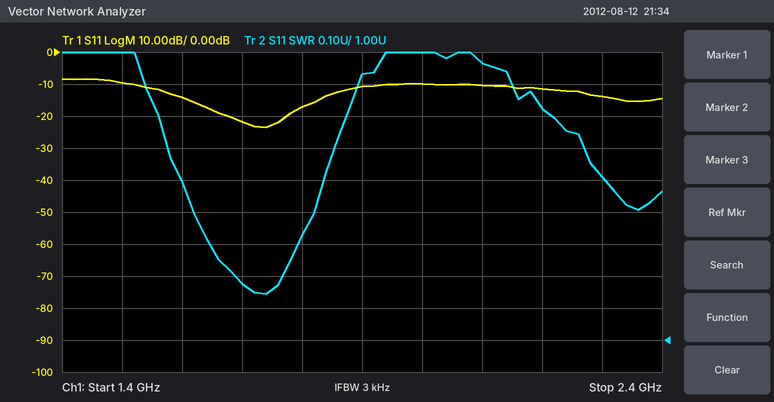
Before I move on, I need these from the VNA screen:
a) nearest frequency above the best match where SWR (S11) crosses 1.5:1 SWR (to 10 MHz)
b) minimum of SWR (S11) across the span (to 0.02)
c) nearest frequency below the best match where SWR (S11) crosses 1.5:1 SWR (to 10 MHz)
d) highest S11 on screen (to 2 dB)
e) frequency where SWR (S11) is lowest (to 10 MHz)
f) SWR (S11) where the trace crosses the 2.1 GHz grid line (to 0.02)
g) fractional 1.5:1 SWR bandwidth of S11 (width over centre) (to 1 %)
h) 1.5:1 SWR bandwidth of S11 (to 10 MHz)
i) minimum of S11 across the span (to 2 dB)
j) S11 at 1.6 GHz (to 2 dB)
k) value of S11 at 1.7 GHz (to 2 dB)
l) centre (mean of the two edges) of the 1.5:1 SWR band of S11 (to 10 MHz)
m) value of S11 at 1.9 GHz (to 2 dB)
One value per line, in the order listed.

1.84 GHz
1.14
1.60 GHz
-8 dB
1.74 GHz
1.86
14 %
240 MHz
-24 dB
-14 dB
-22 dB
1.72 GHz
-10 dB
